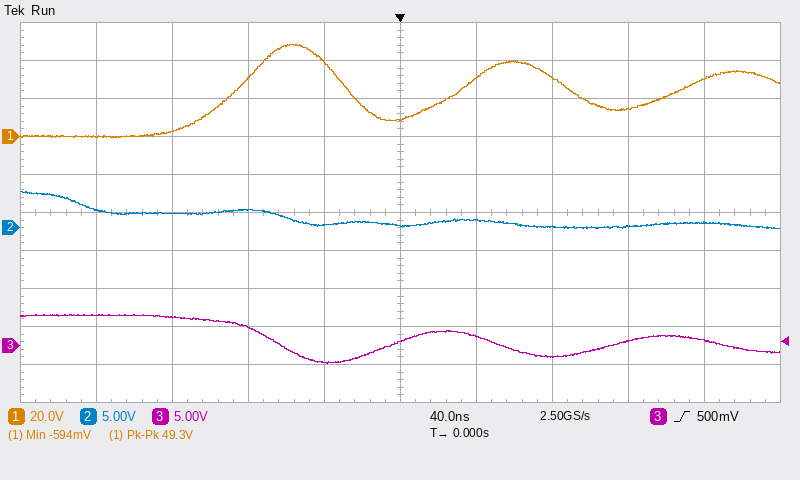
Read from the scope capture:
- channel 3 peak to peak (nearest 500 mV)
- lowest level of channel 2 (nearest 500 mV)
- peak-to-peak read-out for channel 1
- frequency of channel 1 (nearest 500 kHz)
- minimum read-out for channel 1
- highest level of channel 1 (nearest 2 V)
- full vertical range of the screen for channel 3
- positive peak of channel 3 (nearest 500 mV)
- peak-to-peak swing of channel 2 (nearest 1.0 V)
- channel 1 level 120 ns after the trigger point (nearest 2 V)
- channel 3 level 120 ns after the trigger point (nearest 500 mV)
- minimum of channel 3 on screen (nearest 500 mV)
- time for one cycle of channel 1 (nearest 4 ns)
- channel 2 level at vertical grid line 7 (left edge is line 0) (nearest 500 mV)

6.5 V
0.0 V
49.3 V
8.5 MHz
-594 mV
48 V
50 V
4.0 V
5.0 V
14 V
500 mV
-2.5 V
116 ns
0.0 V
